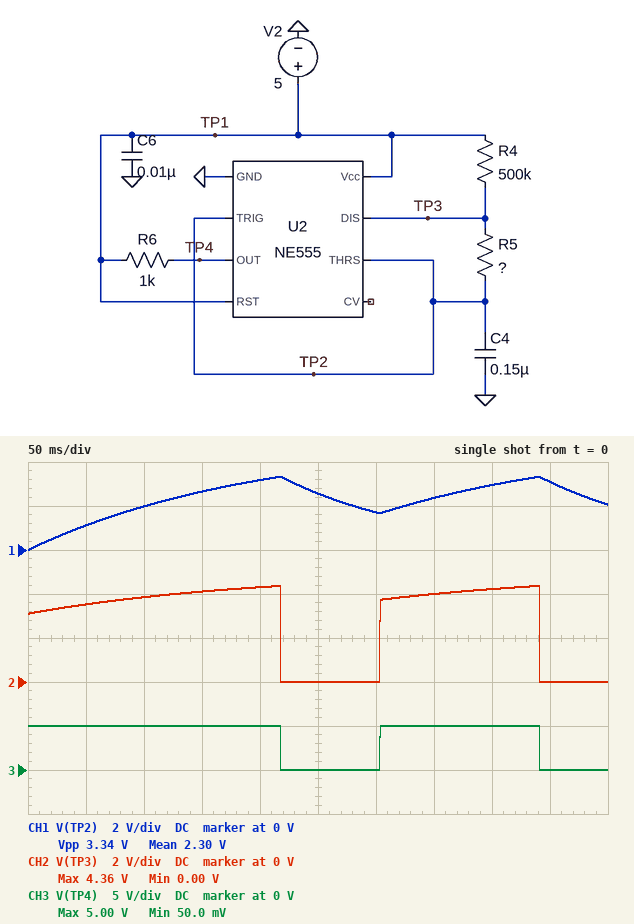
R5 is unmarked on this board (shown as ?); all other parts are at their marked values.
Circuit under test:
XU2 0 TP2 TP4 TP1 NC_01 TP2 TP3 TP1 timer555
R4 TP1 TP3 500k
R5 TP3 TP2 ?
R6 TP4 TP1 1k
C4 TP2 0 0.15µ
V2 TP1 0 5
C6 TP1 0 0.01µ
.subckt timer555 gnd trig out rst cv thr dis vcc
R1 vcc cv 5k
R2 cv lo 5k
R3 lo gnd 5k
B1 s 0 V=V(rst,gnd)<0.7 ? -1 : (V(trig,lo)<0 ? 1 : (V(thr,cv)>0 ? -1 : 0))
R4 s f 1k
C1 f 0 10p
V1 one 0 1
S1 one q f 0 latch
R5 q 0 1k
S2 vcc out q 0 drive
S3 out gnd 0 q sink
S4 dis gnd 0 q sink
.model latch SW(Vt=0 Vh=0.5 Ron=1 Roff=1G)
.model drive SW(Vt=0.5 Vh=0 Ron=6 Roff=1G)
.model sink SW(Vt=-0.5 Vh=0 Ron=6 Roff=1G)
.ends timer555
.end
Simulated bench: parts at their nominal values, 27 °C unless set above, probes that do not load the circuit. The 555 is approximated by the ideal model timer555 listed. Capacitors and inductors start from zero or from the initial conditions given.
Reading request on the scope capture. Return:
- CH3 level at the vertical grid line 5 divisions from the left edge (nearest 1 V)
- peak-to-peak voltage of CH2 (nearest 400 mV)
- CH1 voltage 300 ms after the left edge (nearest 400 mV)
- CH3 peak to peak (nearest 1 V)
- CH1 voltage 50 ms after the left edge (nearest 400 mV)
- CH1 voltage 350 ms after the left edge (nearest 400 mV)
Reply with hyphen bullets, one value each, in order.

- 0 V
- 4.4 V
- 1.6 V
- 5 V
- 1.2 V
- 2.4 V
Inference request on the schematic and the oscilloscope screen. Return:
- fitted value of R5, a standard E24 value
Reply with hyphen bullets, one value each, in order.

- 820 kΩ
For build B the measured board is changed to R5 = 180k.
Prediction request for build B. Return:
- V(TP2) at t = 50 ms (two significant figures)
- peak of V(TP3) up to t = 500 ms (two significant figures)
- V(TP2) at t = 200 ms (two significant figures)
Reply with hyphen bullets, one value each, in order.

- 1.9 V
- 3.8 V
- 3.3 V
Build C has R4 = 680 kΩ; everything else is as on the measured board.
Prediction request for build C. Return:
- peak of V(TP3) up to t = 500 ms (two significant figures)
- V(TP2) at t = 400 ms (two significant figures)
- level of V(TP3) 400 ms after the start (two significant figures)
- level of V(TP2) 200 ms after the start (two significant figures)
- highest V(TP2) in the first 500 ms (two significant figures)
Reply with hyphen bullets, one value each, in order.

- 4.2 V
- 2.5 V
- 3.9 V
- 2.9 V
- 3.3 V
